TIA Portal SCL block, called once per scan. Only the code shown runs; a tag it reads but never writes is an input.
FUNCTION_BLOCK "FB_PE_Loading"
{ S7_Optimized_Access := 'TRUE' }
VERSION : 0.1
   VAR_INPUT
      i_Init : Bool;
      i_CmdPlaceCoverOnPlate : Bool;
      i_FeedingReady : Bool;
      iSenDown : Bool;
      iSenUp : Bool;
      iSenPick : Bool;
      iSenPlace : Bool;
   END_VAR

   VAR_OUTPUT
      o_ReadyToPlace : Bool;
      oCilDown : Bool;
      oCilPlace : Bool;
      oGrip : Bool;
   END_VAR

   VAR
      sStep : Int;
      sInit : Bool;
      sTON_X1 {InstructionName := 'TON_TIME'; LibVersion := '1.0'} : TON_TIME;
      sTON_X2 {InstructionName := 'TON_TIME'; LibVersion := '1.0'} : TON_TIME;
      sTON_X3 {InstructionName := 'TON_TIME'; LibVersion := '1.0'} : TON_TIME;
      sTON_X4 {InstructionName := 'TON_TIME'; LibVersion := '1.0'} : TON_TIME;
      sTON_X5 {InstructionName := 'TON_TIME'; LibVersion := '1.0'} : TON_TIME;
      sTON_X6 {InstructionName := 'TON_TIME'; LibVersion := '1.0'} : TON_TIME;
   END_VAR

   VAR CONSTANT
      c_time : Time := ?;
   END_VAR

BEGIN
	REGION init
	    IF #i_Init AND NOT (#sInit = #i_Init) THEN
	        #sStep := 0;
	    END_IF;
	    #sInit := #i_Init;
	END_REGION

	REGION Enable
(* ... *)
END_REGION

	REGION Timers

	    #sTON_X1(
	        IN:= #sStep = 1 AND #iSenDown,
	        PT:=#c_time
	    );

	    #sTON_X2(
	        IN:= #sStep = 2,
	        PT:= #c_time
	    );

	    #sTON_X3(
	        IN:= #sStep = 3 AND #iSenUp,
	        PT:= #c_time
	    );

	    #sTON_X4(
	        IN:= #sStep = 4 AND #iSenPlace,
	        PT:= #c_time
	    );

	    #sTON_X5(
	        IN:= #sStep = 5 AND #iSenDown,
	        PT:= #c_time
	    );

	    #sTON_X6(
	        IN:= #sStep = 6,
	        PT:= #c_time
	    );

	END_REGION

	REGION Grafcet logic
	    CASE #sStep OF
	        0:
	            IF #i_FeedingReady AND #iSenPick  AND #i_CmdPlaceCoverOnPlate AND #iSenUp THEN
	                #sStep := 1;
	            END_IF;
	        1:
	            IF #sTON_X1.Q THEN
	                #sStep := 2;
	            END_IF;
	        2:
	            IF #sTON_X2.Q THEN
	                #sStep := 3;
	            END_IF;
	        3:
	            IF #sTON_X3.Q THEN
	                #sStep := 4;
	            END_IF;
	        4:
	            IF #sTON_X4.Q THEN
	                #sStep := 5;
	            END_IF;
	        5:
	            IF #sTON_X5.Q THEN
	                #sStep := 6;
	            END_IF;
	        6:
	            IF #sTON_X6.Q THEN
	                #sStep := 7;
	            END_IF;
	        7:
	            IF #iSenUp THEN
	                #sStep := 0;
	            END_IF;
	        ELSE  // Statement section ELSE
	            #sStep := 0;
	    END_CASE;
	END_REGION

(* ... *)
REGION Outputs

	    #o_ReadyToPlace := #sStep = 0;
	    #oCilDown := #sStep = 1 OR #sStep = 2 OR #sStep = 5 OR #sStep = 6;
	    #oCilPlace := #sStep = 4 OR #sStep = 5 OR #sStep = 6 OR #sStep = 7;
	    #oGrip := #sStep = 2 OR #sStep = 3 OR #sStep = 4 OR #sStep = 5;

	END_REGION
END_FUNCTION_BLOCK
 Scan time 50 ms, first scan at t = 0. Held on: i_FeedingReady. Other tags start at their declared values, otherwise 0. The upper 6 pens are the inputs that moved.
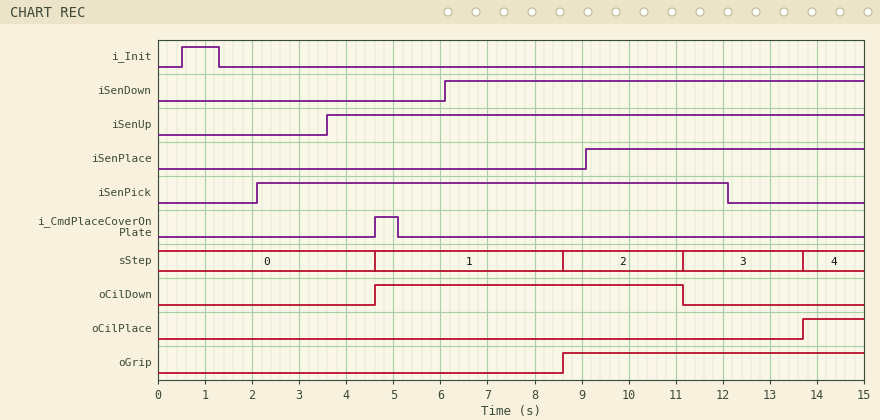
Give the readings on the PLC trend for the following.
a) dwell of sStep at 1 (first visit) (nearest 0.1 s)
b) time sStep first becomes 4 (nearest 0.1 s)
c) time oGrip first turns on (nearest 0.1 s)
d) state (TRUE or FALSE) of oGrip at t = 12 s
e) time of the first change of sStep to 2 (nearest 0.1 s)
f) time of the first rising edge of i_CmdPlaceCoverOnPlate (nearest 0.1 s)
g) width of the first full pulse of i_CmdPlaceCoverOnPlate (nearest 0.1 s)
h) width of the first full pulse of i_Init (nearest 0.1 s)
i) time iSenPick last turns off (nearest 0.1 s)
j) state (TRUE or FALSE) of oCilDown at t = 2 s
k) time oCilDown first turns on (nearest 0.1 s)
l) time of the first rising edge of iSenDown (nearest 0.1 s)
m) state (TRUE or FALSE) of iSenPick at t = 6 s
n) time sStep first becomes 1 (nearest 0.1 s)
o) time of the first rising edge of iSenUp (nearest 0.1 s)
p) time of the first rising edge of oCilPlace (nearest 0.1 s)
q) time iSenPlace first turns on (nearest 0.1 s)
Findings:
4.0 s
13.7 s
8.6 s
TRUE
8.6 s
4.6 s
0.5 s
0.8 s
12.1 s
FALSE
4.6 s
6.1 s
TRUE
4.6 s
3.6 s
13.7 s
9.1 s
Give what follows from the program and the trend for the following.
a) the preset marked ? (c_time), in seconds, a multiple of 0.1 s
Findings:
2.5 s
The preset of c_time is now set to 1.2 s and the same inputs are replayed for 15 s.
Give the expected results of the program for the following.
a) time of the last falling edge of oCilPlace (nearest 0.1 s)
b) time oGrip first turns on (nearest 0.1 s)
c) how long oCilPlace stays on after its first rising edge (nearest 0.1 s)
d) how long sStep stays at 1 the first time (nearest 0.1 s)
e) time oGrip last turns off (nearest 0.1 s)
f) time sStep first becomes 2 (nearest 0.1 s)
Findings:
13.6 s
7.3 s
3.8 s
2.7 s
12.3 s
7.3 s
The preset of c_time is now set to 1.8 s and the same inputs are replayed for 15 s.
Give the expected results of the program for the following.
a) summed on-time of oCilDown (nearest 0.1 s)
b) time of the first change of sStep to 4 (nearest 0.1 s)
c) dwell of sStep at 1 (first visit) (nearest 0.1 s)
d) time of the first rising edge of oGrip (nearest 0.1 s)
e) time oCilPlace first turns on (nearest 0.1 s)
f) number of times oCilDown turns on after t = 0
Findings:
6.7 s
11.6 s
3.3 s
7.9 s
11.6 s
2
